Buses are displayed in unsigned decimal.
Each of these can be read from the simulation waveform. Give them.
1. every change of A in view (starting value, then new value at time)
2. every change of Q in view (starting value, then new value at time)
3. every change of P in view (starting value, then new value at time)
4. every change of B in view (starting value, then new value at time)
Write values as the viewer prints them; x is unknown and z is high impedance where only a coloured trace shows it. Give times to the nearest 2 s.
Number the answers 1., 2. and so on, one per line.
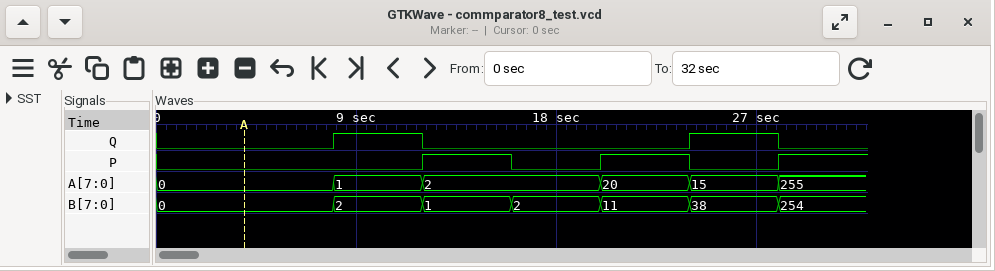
1. 0, 1 at 8 s, 2 at 12 s, 20 at 20 s, 15 at 24 s, 255 at 28 s
2. 0, 1 at 8 s, 0 at 12 s, 1 at 24 s, 0 at 28 s
3. 0, 1 at 12 s, 0 at 16 s, 1 at 20 s, 0 at 24 s, 1 at 28 s
4. 0, 2 at 8 s, 1 at 12 s, 2 at 16 s, 11 at 20 s, 38 at 24 s, 254 at 28 s
